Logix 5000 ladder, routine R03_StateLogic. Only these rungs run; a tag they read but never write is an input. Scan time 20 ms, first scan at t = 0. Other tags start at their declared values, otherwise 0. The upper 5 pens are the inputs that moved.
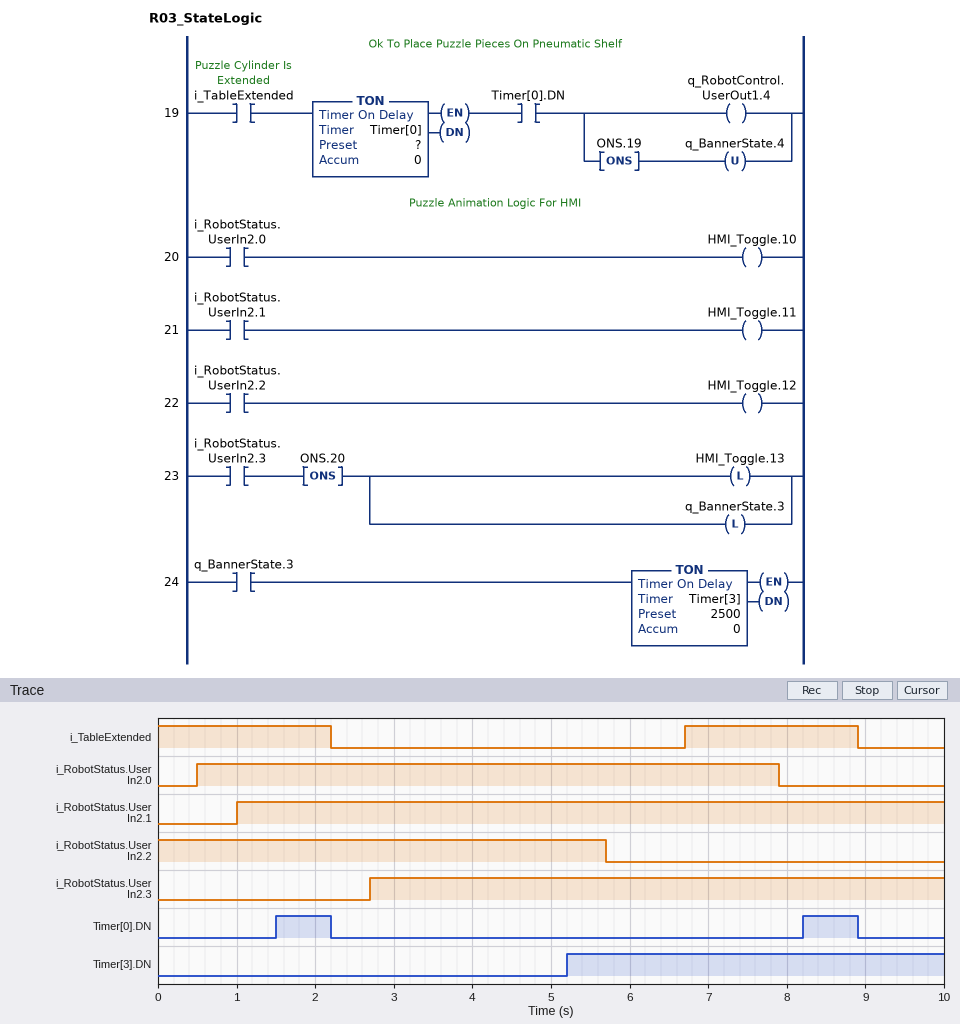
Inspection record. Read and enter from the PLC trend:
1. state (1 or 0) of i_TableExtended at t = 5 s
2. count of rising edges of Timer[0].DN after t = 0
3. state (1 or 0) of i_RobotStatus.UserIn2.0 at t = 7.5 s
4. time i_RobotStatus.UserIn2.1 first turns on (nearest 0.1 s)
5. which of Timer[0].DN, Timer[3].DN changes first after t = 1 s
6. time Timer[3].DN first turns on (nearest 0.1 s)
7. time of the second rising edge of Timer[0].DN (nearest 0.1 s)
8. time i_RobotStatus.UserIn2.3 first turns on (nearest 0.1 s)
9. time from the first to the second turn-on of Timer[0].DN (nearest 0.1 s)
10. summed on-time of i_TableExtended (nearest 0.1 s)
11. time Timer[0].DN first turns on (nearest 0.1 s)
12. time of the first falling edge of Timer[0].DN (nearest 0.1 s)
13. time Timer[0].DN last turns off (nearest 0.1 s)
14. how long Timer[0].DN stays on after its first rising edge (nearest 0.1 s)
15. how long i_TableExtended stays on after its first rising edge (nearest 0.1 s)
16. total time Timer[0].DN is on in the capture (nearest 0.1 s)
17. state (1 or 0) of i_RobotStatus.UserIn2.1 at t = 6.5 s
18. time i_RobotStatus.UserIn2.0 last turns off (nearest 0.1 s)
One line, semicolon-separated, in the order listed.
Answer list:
0; 2; 1; 1.0 s; Timer[0].DN; 5.2 s; 8.2 s; 2.7 s; 6.7 s; 4.4 s; 1.5 s; 2.2 s; 8.9 s; 0.7 s; 2.2 s; 1.4 s; 1; 7.9 s
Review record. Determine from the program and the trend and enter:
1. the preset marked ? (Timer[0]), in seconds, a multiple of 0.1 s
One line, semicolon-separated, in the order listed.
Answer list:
1.5 s
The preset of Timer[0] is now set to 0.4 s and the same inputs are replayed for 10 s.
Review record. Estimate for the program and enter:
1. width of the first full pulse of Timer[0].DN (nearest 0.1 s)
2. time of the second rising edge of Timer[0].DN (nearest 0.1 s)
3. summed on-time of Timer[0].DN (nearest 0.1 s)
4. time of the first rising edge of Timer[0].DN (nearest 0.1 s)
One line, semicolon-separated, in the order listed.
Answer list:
1.8 s; 7.1 s; 3.6 s; 0.4 s
